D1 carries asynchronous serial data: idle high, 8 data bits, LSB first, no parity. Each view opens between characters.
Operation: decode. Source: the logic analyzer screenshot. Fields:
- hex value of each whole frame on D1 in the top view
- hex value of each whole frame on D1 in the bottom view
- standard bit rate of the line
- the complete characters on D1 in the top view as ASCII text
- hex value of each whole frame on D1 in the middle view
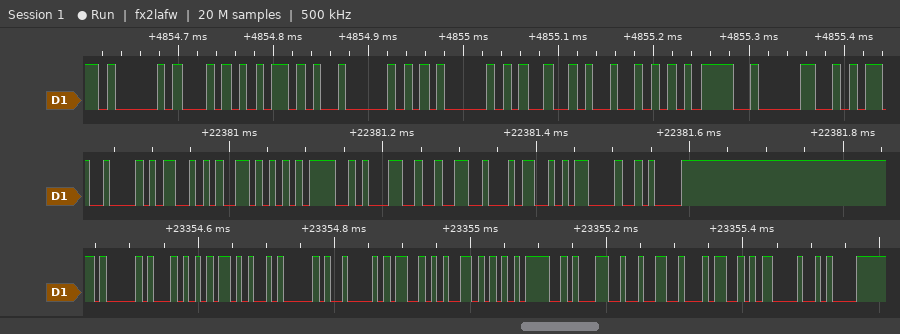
41, 54, 2B, 50, 41, 49, 52, 3D, 30
41, 54, 2B, 41, 42, 53, 56, 3D, 31, 32, 34, 0D, 0A
115200 baud
"AT+PAIR=0"
42, 53, 56, 3D, 31, 32, 34, 0D, 0A
